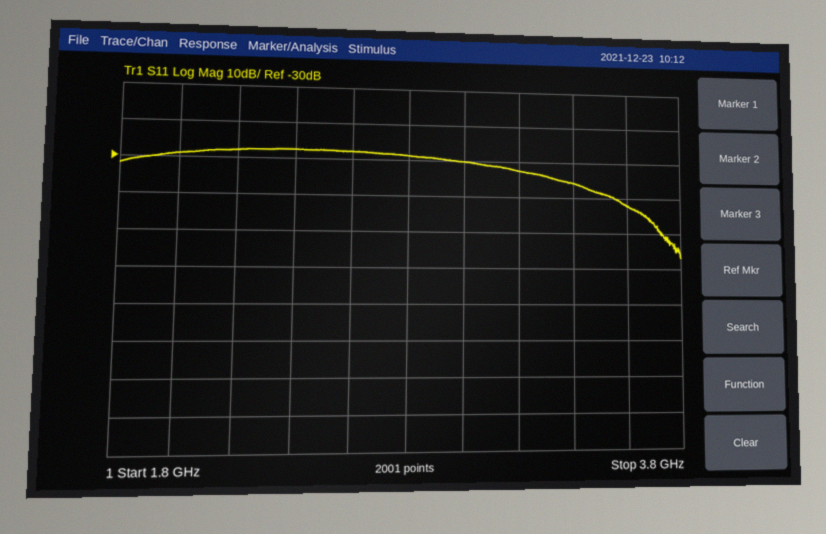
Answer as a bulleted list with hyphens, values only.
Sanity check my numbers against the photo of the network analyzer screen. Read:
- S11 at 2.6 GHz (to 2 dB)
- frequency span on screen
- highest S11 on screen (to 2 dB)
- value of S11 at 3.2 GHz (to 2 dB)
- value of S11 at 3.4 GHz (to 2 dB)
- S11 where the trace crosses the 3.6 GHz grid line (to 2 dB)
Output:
- -28 dB
- 2 GHz
- -28 dB
- -32 dB
- -36 dB
- -42 dB
